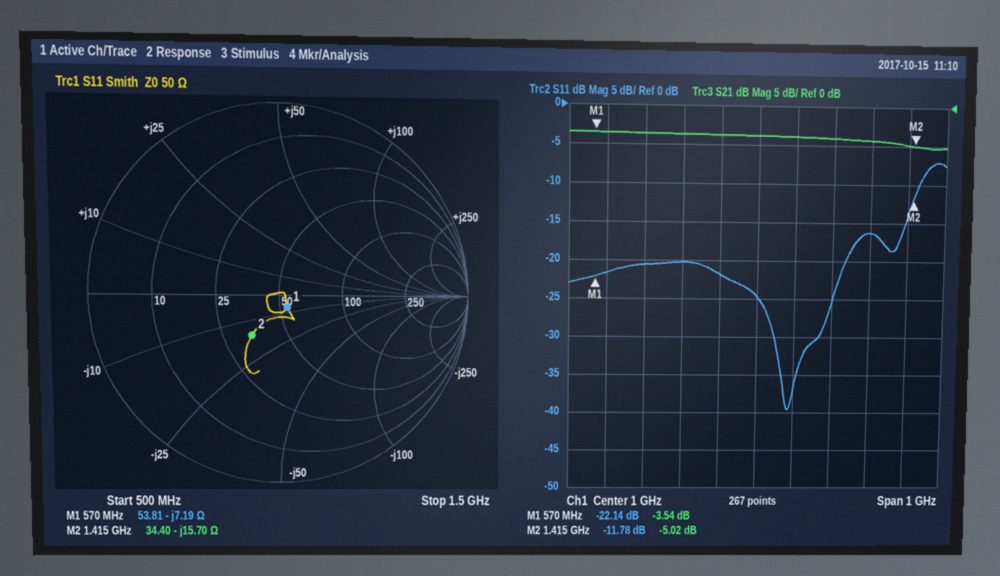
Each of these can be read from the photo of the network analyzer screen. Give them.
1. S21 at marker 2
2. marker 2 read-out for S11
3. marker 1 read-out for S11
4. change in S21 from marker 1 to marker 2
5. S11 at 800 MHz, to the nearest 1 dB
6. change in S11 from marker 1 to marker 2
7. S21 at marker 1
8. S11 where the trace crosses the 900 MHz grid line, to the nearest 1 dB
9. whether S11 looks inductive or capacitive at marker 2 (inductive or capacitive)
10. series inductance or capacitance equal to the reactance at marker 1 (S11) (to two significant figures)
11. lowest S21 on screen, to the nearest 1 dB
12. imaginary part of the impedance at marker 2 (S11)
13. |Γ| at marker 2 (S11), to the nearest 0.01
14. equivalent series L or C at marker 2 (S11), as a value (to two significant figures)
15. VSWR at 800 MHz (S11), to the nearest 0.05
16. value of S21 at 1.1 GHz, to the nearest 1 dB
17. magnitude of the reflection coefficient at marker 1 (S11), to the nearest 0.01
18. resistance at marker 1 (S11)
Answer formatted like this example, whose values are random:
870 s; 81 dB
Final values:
-5.02 dB; -11.78 dB; -22.14 dB; -1.48 dB; -20 dB; 10.36 dB; -3.54 dB; -22 dB; capacitive; 39 pF; -5 dB; -15.70 Ω; 0.26; 7.2 pF; 1.20; -4 dB; 0.08; 53.81 Ω
